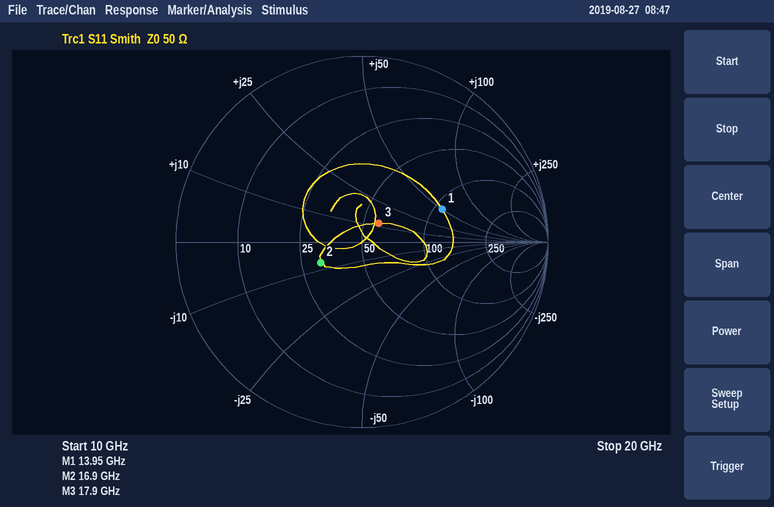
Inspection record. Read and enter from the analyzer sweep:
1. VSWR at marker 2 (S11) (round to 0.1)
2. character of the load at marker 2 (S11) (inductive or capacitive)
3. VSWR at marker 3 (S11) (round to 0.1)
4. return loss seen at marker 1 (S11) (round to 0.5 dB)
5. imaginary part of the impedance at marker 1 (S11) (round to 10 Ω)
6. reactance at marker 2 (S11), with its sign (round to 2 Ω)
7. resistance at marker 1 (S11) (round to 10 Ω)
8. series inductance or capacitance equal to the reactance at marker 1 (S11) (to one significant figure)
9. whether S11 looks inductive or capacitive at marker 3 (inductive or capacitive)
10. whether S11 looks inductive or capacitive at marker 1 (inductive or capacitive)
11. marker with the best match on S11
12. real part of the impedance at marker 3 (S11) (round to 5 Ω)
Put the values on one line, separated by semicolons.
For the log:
1.7; capacitive; 1.3; 6.5 dB; +50 Ω; -8 Ω; 110 Ω; 600 pH; inductive; inductive; marker 3; 60 Ω
